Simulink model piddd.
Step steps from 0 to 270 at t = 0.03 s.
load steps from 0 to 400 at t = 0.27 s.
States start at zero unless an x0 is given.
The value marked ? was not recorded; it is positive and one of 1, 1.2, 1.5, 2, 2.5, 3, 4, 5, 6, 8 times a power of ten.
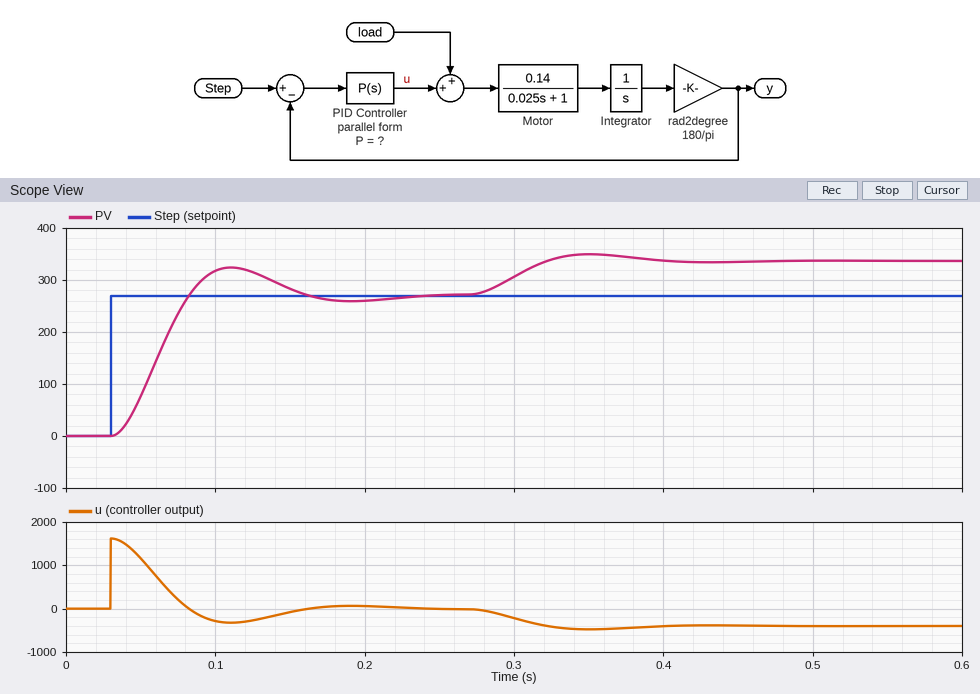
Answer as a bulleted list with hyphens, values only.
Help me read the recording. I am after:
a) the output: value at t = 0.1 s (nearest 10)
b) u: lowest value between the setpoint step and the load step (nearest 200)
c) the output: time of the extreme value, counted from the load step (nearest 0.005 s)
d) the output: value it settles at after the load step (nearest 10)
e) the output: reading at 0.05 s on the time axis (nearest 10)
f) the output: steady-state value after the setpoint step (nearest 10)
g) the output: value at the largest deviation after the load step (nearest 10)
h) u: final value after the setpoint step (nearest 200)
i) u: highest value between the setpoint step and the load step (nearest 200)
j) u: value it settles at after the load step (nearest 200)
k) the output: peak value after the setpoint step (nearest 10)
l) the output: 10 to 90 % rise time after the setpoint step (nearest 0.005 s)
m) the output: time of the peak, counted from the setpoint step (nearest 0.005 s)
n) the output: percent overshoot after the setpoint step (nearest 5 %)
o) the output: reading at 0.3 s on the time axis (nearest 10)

- 320
- -400
- 0.080 s
- 340
- 80
- 270
- 350
- 0
- 1600
- -400
- 320
- 0.035 s
- 0.080 s
- 20 %
- 310
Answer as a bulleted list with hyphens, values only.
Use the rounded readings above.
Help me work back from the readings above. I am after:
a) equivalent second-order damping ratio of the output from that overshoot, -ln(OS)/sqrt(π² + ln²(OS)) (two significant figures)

- 0.46
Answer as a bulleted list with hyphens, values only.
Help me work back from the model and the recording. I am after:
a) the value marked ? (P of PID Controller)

- 6
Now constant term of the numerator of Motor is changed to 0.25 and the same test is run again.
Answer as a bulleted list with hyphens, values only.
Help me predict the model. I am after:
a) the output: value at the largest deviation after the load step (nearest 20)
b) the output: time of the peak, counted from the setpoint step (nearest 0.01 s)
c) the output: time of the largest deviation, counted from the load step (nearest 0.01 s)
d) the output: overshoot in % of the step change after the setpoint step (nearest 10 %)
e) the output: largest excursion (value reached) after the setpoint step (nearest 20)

- 360
- 0.06 s
- 0.06 s
- 30 %
- 360
